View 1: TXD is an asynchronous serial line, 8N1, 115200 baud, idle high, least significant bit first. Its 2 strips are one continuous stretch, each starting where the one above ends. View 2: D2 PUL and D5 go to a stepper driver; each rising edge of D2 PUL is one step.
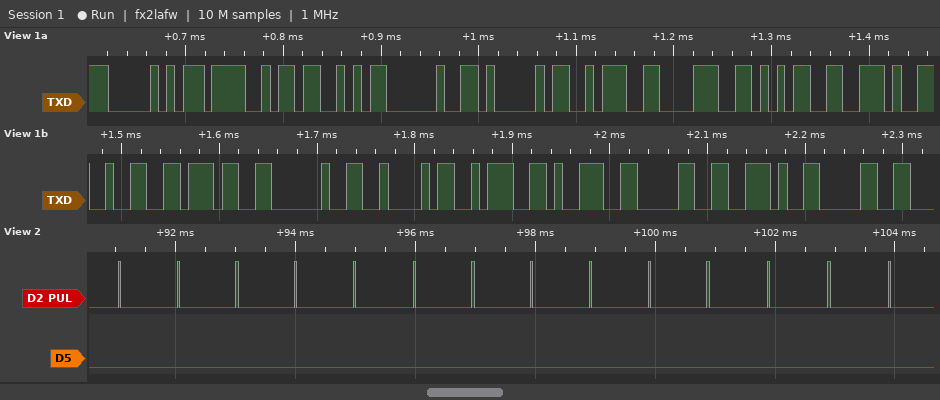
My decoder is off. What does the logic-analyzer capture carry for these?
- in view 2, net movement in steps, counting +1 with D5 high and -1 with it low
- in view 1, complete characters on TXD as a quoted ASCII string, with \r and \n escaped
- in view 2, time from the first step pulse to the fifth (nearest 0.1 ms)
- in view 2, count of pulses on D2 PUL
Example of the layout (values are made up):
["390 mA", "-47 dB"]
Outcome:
["-14", "\"POS A:85.27 B:90.0\"", "3.9 ms", "14"]
